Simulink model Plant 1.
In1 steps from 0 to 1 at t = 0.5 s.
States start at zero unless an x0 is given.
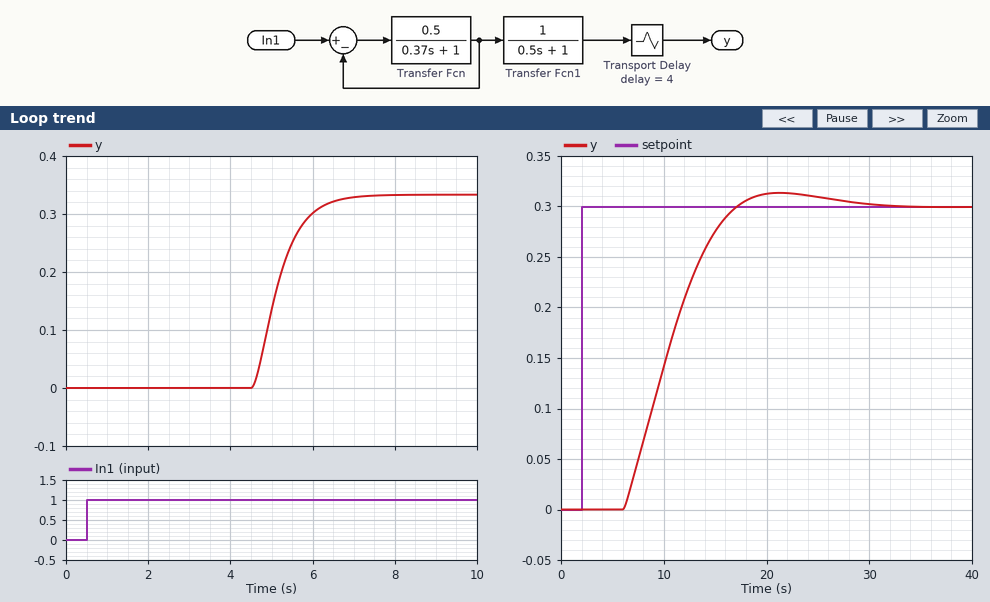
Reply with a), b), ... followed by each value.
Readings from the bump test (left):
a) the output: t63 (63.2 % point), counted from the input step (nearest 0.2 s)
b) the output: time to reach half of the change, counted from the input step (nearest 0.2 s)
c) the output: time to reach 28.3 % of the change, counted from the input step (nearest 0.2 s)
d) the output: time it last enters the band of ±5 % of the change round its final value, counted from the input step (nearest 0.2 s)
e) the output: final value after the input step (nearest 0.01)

a) 4.8 s
b) 4.6 s
c) 4.4 s
d) 5.8 s
e) 0.33
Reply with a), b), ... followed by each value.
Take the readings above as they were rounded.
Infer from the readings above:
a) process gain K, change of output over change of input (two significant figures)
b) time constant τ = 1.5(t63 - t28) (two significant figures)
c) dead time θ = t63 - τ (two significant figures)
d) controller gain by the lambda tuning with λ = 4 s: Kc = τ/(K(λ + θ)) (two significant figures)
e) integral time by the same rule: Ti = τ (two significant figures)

a) 0.33
b) 0.60 s
c) 4.2 s
d) 0.22
e) 0.60 s
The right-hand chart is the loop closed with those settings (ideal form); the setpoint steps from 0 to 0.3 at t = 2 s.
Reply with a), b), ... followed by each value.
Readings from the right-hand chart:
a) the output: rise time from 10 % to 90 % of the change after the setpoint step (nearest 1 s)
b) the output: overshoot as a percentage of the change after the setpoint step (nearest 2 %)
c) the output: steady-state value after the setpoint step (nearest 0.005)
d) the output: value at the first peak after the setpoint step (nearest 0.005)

a) 8 s
b) 4 %
c) 0.300
d) 0.315
